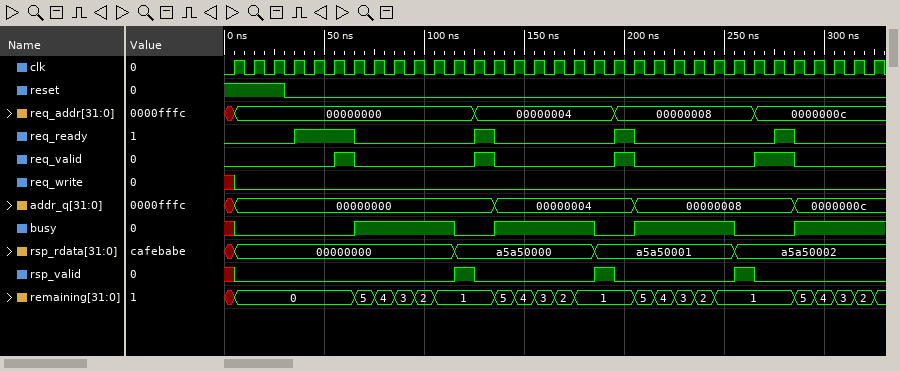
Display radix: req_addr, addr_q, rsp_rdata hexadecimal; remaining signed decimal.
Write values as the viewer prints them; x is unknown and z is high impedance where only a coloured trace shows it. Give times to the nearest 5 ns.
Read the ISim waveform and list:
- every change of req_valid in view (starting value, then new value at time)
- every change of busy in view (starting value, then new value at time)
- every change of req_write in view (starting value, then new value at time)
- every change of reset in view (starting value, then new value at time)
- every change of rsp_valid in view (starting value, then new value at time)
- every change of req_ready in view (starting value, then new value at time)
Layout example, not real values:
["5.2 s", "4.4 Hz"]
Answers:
["0, 1 at 55 ns, 0 at 65 ns, 1 at 125 ns, 0 at 135 ns, 1 at 195 ns, 0 at 205 ns, 1 at 265 ns, 0 at 285 ns", "x, 0 at 5 ns, 1 at 65 ns, 0 at 115 ns, 1 at 135 ns, 0 at 185 ns, 1 at 205 ns, 0 at 255 ns, 1 at 285 ns", "x, 0 at 5 ns", "1, 0 at 30 ns", "x, 0 at 5 ns, 1 at 115 ns, 0 at 125 ns, 1 at 185 ns, 0 at 195 ns, 1 at 255 ns, 0 at 265 ns", "0, 1 at 35 ns, 0 at 65 ns, 1 at 125 ns, 0 at 135 ns, 1 at 195 ns, 0 at 205 ns, 1 at 275 ns, 0 at 285 ns"]
